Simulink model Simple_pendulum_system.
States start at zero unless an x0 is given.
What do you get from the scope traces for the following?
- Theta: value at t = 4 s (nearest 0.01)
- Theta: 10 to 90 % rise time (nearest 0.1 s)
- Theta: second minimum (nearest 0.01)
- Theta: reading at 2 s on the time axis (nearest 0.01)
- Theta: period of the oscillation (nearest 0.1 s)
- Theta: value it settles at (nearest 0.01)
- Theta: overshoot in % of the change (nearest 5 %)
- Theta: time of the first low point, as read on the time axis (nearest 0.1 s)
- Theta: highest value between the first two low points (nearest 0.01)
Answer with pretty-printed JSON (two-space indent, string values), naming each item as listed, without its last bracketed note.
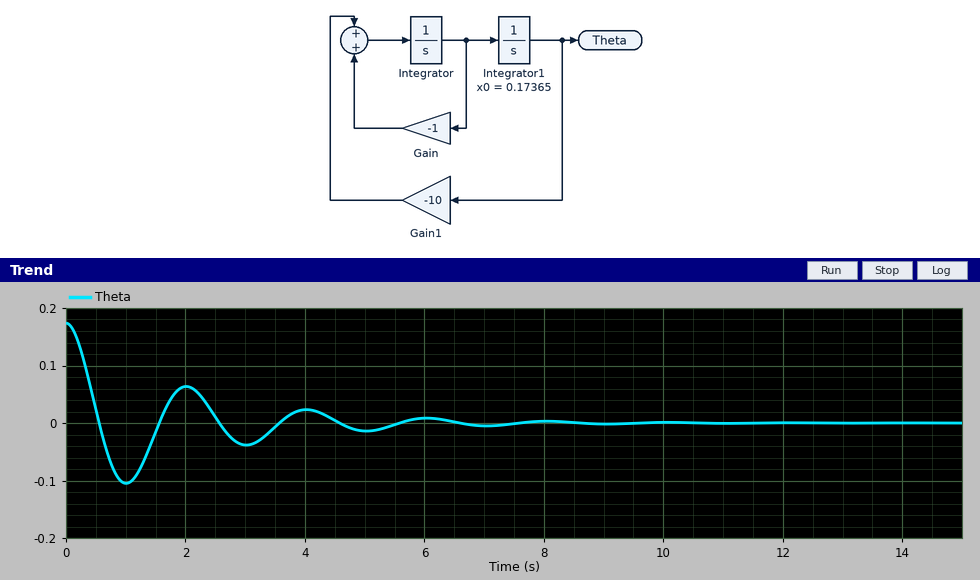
{
  "Theta: value at t = 4 s": "0.02",
  "Theta: 10 to 90 % rise time": "0.4 s",
  "Theta: second minimum": "-0.04",
  "Theta: reading at 2 s on the time axis": "0.06",
  "Theta: period of the oscillation": "2.0 s",
  "Theta: value it settles at": "0.00",
  "Theta: overshoot in % of the change": "60 %",
  "Theta: time of the first low point, as read on the time axis": "1.0 s",
  "Theta: highest value between the first two low points": "0.06"
}
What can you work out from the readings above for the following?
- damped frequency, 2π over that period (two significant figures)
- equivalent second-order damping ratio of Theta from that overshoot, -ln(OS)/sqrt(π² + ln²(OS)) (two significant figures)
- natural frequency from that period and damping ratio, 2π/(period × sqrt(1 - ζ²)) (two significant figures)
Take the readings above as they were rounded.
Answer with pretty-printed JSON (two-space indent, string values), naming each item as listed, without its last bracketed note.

{
  "damped frequency, 2π over that period": "3.1 rad/s",
  "equivalent second-order damping ratio of Theta from that overshoot, -ln(OS)/sqrt(π² + ln²(OS))": "0.16",
  "natural frequency from that period and damping ratio, 2π/(period × sqrt(1 - ζ²))": "3.2 rad/s"
}
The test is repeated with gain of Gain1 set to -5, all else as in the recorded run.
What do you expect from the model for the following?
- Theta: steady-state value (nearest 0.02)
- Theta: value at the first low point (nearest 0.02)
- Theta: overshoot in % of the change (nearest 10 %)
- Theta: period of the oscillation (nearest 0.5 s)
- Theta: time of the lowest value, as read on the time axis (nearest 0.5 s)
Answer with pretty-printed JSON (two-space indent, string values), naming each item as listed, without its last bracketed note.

{
  "Theta: steady-state value": "0.00",
  "Theta: value at the first low point": "-0.08",
  "Theta: overshoot in % of the change": "50 %",
  "Theta: period of the oscillation": "3.0 s",
  "Theta: time of the lowest value, as read on the time axis": "1.5 s"
}
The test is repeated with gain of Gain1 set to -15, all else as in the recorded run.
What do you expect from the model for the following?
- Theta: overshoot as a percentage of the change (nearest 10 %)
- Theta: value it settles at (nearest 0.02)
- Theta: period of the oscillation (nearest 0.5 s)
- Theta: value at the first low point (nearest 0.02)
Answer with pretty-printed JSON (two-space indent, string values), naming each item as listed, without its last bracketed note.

{
  "Theta: overshoot as a percentage of the change": "70 %",
  "Theta: value it settles at": "0.00",
  "Theta: period of the oscillation": "1.5 s",
  "Theta: value at the first low point": "-0.12"
}
